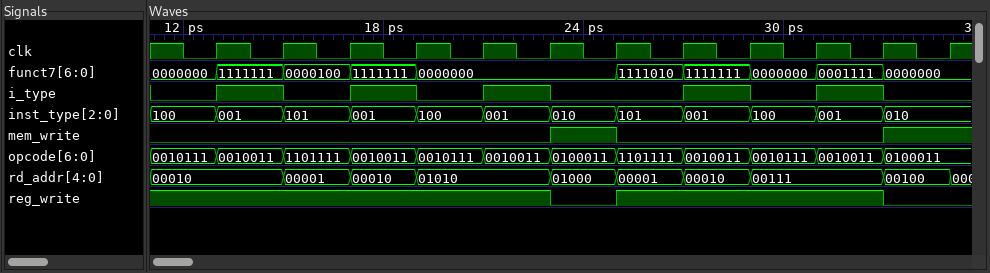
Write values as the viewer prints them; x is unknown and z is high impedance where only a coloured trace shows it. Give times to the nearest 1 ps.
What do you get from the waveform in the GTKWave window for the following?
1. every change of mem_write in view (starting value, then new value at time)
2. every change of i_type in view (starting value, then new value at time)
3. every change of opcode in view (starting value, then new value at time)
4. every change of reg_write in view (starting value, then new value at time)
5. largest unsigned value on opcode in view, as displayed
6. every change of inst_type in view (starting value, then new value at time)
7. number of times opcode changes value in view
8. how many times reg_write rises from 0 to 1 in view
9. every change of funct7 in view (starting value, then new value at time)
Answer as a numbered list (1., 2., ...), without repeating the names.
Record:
1. 0, 1 at 23 ps, 0 at 25 ps, 1 at 33 ps
2. 0, 1 at 13 ps, 0 at 15 ps, 1 at 17 ps, 0 at 19 ps, 1 at 21 ps, 0 at 23 ps, 1 at 27 ps, 0 at 29 ps, 1 at 31 ps, 0 at 33 ps
3. 0010111, 0010011 at 13 ps, 1101111 at 15 ps, 0010011 at 17 ps, 0010111 at 19 ps, 0010011 at 21 ps, 0100011 at 23 ps, 1101111 at 25 ps, 0010011 at 27 ps, 0010111 at 29 ps, 0010011 at 31 ps, 0100011 at 33 ps
4. 1, 0 at 23 ps, 1 at 25 ps, 0 at 33 ps
5. 1101111
6. 100, 001 at 13 ps, 101 at 15 ps, 001 at 17 ps, 100 at 19 ps, 001 at 21 ps, 010 at 23 ps, 101 at 25 ps, 001 at 27 ps, 100 at 29 ps, 001 at 31 ps, 010 at 33 ps
7. 11
8. 1
9. 0000000, 1111111 at 13 ps, 0000100 at 15 ps, 1111111 at 17 ps, 0000000 at 19 ps, 1111010 at 25 ps, 1111111 at 27 ps, 0000000 at 29 ps, 0001111 at 31 ps, 0000000 at 33 ps
